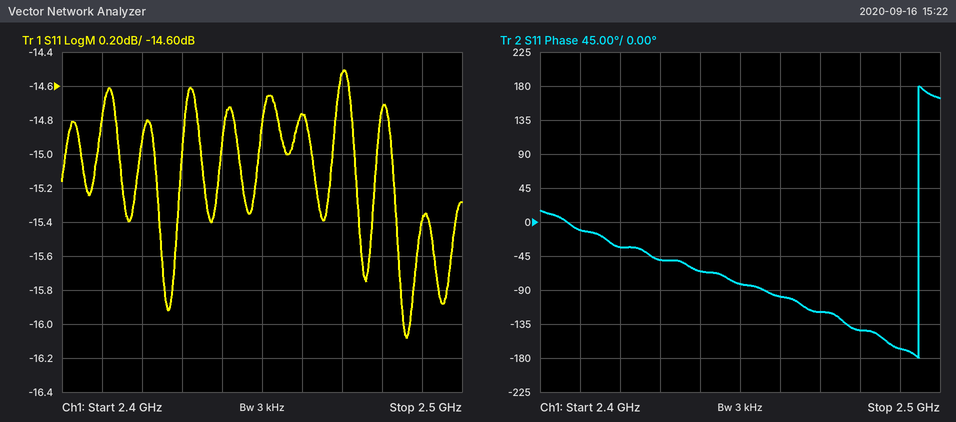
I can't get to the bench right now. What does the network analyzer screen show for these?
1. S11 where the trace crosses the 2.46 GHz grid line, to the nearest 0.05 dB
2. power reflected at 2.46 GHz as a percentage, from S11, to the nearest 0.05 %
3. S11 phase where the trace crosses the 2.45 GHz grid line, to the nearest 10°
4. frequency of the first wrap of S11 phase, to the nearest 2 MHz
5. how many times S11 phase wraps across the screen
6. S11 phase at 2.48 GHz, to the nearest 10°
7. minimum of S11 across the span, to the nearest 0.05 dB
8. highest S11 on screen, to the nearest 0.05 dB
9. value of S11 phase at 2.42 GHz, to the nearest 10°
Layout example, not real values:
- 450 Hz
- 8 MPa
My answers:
- -14.75 dB
- 3.35 %
- -80°
- 2.494 GHz
- 1
- -140°
- -16.10 dB
- -14.50 dB
- -30°
